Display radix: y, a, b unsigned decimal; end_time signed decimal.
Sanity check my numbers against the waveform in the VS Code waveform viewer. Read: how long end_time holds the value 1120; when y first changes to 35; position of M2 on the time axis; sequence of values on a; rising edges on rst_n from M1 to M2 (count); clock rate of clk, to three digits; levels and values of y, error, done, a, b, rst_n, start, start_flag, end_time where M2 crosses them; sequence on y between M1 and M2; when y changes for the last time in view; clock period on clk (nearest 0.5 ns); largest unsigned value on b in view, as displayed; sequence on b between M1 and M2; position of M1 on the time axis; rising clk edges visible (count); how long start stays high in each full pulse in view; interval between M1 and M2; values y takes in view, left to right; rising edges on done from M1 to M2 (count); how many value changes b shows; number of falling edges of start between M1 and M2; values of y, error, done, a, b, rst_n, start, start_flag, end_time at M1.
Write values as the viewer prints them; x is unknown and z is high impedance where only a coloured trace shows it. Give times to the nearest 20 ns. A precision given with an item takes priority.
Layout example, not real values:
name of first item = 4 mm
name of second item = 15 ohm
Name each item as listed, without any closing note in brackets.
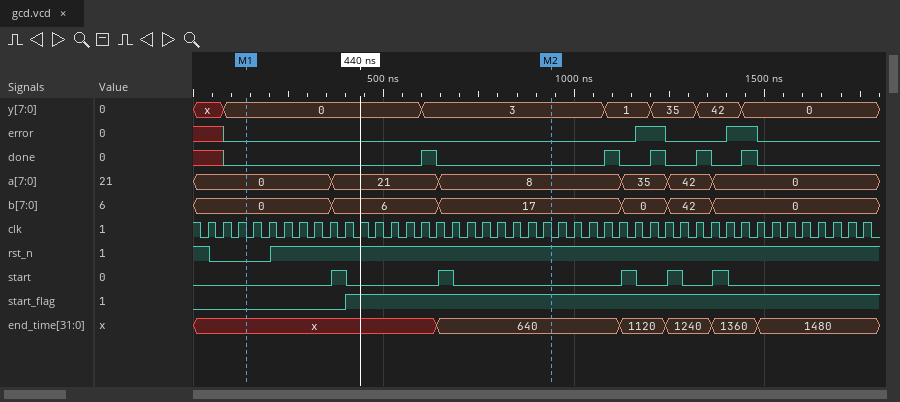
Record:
how long end_time holds the value 1120 = 120 ns
when y first changes to 35 = 1200 ns
position of M2 on the time axis = 940 ns
sequence of values on a = 0, 21, 8, 35, 42, 0
rising edges on rst_n from M1 to M2 = 1
clock rate of clk, to three digits = 25.0 MHz
levels and values of y, error, done, a, b, rst_n, start, start_flag, end_time where M2 crosses them = y=3, error=0, done=0, a=8, b=17, rst_n=1, start=0, start_flag=1, end_time=640
sequence on y between M1 and M2 = 0, 3
when y changes for the last time in view = 1440 ns
clock period on clk = 40 ns
largest unsigned value on b in view, as displayed = 42
sequence on b between M1 and M2 = 0, 6, 17
position of M1 on the time axis = 140 ns
rising clk edges visible = 44
how long start stays high in each full pulse in view = 40 ns, 40 ns, 40 ns, 40 ns, 40 ns
interval between M1 and M2 = 800 ns
values y takes in view, left to right = x, 0, 3, 1, 35, 42, 0
rising edges on done from M1 to M2 = 1
how many value changes b shows = 5
number of falling edges of start between M1 and M2 = 2
values of y, error, done, a, b, rst_n, start, start_flag, end_time at M1 = y=0, error=0, done=0, a=0, b=0, rst_n=0, start=0, start_flag=0, end_time=x
